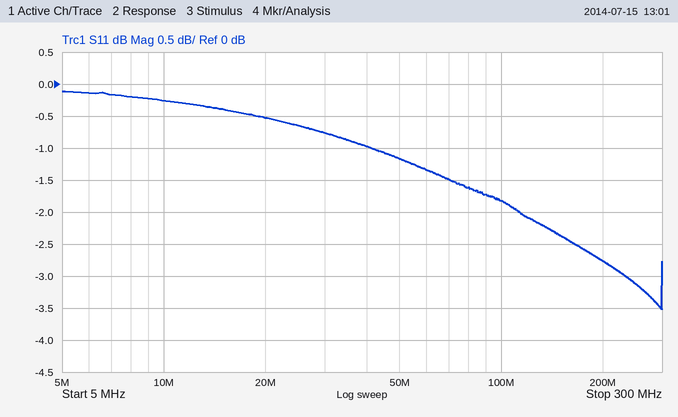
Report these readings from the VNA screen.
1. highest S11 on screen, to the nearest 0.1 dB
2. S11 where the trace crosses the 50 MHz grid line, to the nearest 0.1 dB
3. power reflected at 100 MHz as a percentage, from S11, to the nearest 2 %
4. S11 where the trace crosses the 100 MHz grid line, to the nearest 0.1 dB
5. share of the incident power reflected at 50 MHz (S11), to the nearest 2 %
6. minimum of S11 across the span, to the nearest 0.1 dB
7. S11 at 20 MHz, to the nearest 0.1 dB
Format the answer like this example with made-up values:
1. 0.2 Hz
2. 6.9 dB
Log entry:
1. -0.1 dB
2. -1.2 dB
3. 66 %
4. -1.8 dB
5. 76 %
6. -3.5 dB
7. -0.5 dB
